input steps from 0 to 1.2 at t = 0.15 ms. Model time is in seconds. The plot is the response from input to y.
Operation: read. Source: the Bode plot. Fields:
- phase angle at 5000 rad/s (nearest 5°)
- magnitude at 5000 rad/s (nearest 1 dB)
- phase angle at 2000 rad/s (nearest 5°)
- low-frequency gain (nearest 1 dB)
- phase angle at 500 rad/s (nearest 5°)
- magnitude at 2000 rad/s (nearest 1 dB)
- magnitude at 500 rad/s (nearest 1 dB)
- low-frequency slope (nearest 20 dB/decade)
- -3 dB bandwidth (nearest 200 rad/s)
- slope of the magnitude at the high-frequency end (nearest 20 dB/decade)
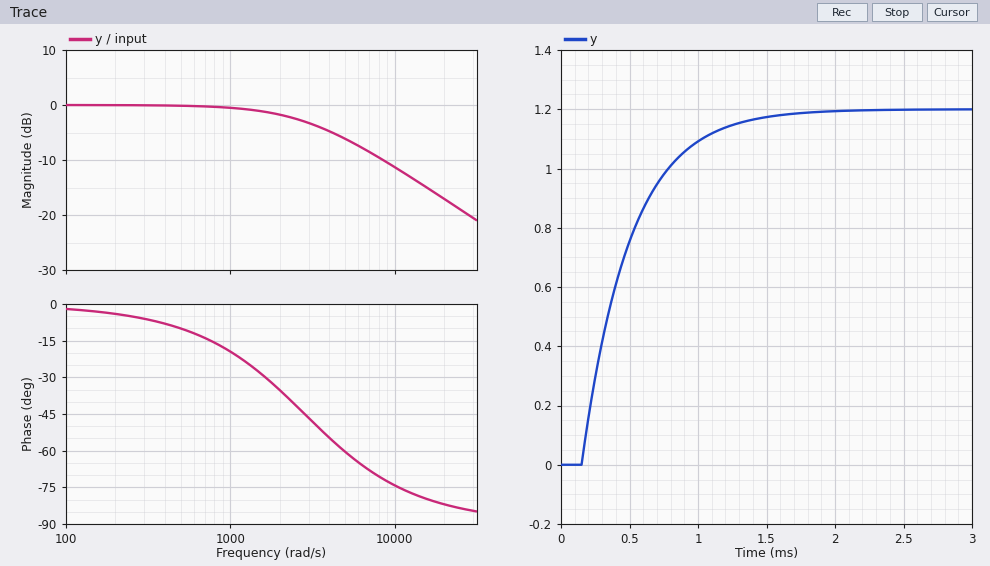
-60°
-6 dB
-35°
0 dB
-10°
-2 dB
0 dB
0 dB/decade
2800 rad/s
-20 dB/decade
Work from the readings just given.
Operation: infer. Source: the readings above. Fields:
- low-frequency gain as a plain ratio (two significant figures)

1.0
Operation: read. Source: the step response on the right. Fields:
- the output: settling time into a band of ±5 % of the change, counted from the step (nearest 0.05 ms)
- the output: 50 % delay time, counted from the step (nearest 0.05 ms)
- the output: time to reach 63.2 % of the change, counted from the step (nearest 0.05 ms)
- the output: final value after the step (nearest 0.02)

1.05 ms
0.25 ms
0.35 ms
1.20
